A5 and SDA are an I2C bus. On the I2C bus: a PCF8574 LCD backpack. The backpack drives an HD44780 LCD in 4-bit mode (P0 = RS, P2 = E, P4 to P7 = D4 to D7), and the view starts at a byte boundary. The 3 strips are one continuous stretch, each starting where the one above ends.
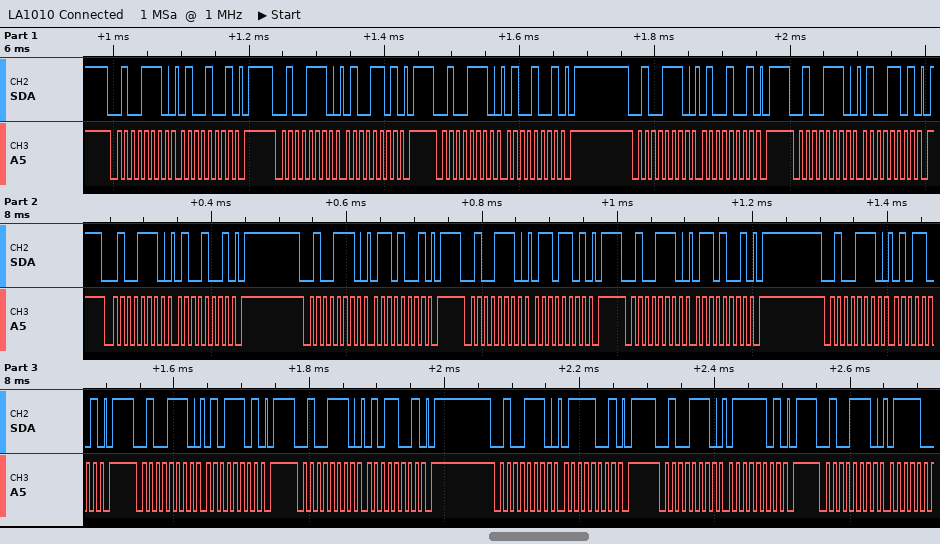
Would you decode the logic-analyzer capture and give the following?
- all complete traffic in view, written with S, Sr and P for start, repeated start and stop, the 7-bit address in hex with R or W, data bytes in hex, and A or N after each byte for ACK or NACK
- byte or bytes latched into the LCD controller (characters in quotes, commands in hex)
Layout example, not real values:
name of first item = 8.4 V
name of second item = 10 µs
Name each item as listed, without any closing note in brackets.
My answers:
all complete traffic in view, written with S, Sr and P for start, repeated start and stop, the 7-bit address in hex with R or W, data bytes in hex, and A or N after each byte for ACK or NACK = S 27W A 49 A P S 27W A 4D A P S 27W A 49 A P S 27W A 49 A P S 27W A 4D A P S 27W A 49 A P S 27W A 69 A P S 27W A 6D A P S 27W A 69 A P S 27W A 59 A P S 27W A 5D A P S 27W A 59 A P S 27W A 79 A P S 27W A 7D A P S 27W A
byte or bytes latched into the LCD controller = 'D' 'e'
